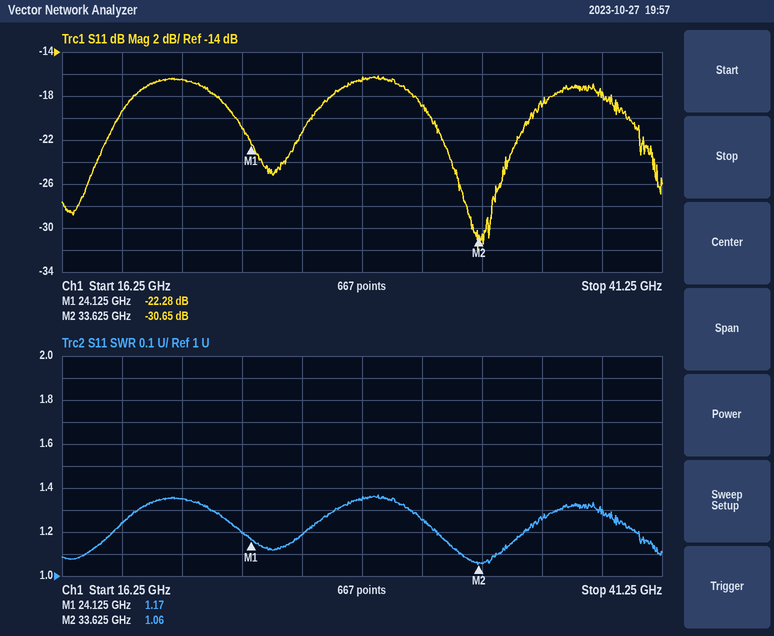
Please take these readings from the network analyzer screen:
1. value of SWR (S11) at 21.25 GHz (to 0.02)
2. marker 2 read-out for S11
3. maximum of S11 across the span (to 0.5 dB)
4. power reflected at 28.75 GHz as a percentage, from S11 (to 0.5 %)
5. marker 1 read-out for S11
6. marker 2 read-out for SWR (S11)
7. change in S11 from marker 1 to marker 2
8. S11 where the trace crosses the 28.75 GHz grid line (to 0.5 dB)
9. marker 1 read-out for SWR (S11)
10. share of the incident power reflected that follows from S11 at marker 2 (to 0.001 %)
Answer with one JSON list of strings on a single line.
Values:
["1.36", "-30.65 dB", "-16.0 dB", "2.0 %", "-22.28 dB", "1.06", "-8.37 dB", "-16.5 dB", "1.17", "0.086 %"]
